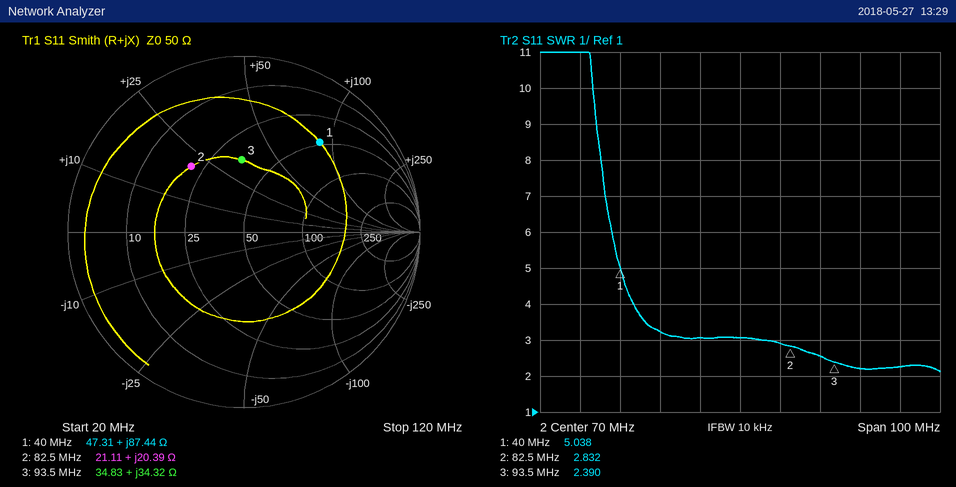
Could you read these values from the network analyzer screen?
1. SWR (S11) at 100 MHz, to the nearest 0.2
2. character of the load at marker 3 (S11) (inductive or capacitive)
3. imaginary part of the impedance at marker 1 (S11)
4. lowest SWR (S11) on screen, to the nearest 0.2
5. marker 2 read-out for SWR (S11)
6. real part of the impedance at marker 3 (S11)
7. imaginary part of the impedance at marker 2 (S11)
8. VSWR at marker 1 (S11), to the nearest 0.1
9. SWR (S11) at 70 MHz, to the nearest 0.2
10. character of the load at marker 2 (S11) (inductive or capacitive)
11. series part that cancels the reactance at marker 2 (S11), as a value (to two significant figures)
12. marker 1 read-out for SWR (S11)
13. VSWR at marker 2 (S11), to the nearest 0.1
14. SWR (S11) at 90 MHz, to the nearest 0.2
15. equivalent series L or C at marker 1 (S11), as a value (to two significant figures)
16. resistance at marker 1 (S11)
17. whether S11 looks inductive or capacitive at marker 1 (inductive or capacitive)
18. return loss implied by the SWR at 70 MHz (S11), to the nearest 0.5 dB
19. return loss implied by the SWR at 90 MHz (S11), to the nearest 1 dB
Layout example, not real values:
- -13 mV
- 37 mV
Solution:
- 2.2
- inductive
- +87.44 Ω
- 2.2
- 2.832
- 34.83 Ω
- +20.39 Ω
- 5.0
- 3.0
- inductive
- 95 pF
- 5.038
- 2.8
- 2.6
- 350 nH
- 47.31 Ω
- inductive
- 6.0 dB
- 7 dB
